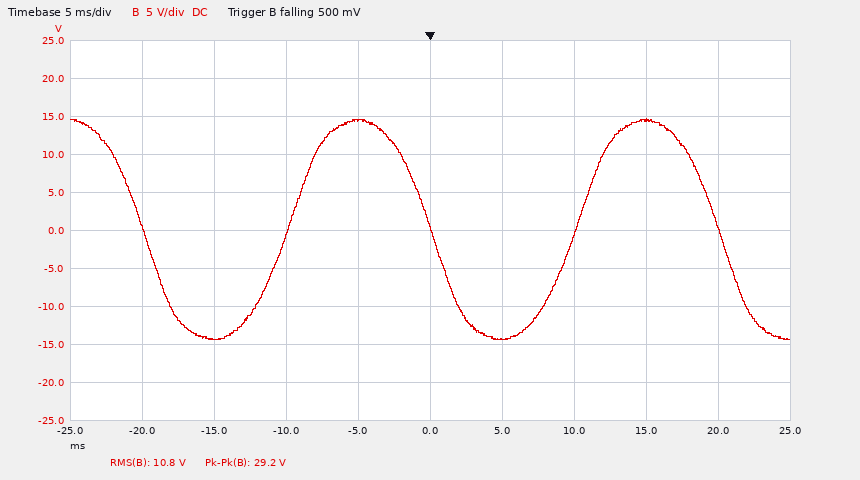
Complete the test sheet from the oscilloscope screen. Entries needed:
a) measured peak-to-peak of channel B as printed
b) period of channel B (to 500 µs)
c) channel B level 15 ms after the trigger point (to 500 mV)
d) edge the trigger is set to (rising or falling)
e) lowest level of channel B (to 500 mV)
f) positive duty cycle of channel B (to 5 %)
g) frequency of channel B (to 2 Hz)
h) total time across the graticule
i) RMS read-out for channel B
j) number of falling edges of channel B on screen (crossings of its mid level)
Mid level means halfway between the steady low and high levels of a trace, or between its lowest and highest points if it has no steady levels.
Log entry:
29.2 V
20.0 ms
14.5 V
falling
-14.5 V
50 %
50 Hz
50 ms
10.8 V
3
